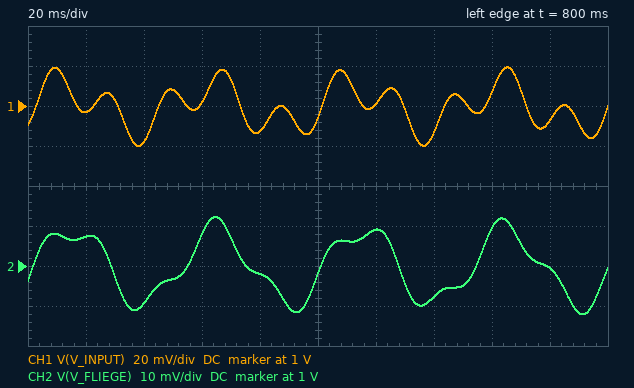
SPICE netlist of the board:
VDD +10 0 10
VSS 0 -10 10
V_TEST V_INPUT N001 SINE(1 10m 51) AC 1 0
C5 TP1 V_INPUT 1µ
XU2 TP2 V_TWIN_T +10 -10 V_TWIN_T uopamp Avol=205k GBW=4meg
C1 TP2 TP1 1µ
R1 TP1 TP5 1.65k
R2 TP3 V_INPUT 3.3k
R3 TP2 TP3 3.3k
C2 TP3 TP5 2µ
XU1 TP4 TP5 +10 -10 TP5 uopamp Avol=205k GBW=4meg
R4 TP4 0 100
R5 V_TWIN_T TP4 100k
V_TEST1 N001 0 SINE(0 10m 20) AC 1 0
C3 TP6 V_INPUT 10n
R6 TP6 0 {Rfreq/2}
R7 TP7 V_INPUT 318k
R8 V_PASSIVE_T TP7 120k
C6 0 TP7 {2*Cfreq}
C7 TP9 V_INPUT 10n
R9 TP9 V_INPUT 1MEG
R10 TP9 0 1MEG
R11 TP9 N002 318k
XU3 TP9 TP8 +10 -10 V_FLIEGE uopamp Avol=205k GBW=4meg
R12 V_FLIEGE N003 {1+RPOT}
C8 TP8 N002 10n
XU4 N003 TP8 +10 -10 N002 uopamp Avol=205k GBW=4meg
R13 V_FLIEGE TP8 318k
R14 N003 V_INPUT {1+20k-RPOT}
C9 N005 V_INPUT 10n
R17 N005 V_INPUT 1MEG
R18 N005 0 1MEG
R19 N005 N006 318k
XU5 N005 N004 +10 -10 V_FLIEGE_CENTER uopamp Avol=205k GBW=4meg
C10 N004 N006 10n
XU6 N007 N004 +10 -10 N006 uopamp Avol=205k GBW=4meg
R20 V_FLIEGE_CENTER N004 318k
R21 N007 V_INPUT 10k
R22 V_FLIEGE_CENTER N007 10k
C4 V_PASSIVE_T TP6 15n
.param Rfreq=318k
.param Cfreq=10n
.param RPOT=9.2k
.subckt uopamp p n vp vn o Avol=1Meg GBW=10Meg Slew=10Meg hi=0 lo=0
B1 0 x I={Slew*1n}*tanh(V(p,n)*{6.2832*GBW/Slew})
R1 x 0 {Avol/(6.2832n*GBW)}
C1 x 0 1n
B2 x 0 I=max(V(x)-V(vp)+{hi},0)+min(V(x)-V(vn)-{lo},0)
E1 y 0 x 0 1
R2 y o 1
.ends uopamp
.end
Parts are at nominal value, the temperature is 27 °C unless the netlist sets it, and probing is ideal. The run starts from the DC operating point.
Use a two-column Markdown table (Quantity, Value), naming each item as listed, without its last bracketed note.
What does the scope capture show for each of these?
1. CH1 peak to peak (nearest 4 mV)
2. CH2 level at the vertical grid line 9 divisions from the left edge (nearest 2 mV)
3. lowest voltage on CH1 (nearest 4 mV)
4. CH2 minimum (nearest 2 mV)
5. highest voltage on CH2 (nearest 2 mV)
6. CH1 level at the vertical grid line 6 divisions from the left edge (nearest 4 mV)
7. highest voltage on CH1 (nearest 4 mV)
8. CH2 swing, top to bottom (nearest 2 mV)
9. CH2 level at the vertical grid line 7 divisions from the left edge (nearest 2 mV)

| Quantity | Value |
|---|---|
| CH1 peak to peak | 40 mV |
| CH2 level at the vertical grid line 9 divisions from the left edge | 1.000 V |
| lowest voltage on CH1 | 980 mV |
| CH2 minimum | 988 mV |
| highest voltage on CH2 | 1.012 V |
| CH1 level at the vertical grid line 6 divisions from the left edge | 1.000 V |
| highest voltage on CH1 | 1.020 V |
| CH2 swing, top to bottom | 24 mV |
| CH2 level at the vertical grid line 7 divisions from the left edge | 992 mV |
